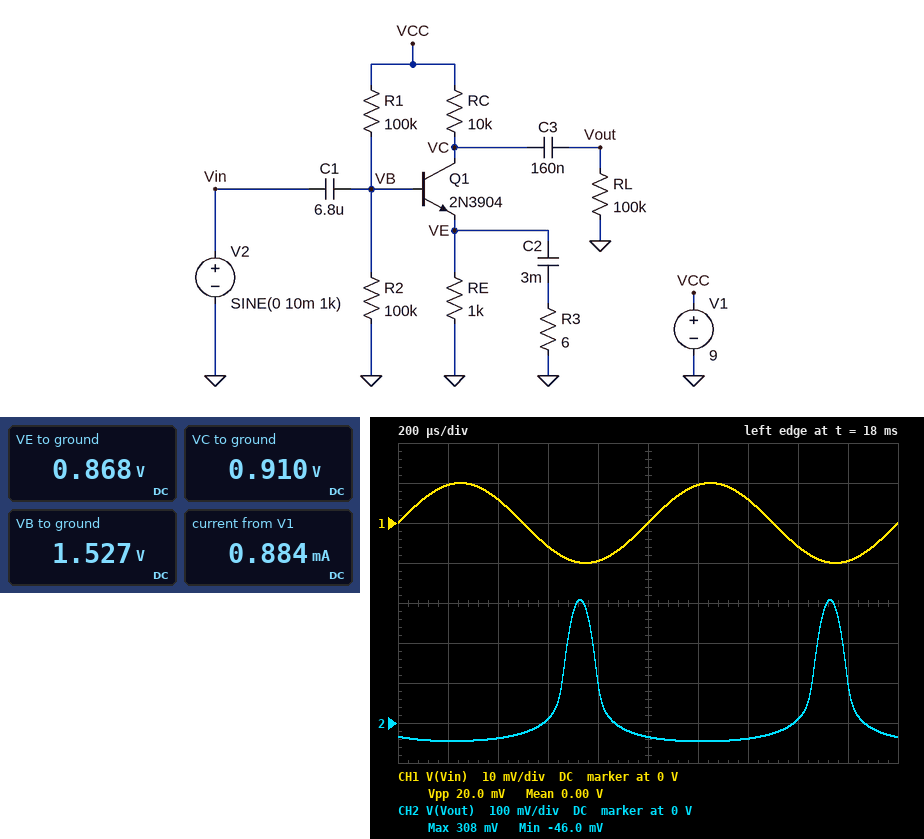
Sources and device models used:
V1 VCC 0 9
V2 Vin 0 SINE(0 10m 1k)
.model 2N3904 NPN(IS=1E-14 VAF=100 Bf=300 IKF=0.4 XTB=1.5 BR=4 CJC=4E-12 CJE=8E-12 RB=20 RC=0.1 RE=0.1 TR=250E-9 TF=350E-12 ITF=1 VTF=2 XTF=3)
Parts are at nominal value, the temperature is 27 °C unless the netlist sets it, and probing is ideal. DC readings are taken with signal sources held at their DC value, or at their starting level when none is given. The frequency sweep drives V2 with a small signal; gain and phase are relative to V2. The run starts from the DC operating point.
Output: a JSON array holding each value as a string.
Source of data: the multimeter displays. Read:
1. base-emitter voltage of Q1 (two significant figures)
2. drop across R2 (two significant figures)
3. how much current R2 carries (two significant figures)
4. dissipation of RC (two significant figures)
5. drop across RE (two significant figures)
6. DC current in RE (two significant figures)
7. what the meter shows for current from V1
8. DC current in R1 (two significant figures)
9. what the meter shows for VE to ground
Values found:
["660 mV", "1.5 V", "15 µA", "6.5 mW", "870 mV", "870 µA", "0.884 mA", "75 µA", "0.868 V"]
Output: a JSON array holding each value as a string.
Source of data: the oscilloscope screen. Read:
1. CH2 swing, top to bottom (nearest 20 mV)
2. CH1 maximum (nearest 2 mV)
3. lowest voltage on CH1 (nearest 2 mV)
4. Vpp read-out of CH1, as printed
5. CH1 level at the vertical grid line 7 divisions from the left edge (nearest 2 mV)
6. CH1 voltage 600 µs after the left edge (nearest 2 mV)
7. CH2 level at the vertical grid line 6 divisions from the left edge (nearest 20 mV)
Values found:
["360 mV", "10 mV", "-10 mV", "20.0 mV", "6 mV", "-6 mV", "-40 mV"]
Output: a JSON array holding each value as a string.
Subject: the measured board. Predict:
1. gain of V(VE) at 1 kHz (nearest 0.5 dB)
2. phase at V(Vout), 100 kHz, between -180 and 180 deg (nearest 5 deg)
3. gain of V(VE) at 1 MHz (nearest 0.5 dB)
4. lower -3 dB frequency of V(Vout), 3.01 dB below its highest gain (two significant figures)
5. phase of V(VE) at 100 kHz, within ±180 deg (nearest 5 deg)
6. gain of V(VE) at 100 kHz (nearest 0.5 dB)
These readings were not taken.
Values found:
["-27.5 dB", "165 deg", "-19.0 dB", "160 Hz", "20 deg", "-26.0 dB"]
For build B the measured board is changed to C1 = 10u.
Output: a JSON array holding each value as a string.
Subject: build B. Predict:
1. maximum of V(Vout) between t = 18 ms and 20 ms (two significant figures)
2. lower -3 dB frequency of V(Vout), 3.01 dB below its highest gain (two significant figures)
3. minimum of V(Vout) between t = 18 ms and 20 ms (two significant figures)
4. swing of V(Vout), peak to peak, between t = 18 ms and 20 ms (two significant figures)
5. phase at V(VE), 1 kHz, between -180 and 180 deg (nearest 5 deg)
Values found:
["320 mV", "110 Hz", "-48 mV", "370 mV", "5 deg"]
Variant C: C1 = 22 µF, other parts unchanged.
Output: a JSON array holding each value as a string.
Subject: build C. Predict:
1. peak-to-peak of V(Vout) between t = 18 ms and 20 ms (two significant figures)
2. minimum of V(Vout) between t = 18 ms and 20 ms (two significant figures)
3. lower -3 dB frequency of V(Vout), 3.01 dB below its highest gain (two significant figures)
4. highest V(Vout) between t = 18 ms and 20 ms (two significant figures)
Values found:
["380 mV", "-48 mV", "53 Hz", "340 mV"]
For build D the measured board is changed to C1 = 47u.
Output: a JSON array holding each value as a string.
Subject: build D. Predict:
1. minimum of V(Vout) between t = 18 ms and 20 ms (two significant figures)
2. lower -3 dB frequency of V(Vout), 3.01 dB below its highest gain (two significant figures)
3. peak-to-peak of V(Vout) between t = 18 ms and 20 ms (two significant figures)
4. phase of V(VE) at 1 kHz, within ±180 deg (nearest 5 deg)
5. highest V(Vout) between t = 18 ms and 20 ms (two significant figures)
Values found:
["-45 mV", "27 Hz", "380 mV", "0 deg", "330 mV"]
